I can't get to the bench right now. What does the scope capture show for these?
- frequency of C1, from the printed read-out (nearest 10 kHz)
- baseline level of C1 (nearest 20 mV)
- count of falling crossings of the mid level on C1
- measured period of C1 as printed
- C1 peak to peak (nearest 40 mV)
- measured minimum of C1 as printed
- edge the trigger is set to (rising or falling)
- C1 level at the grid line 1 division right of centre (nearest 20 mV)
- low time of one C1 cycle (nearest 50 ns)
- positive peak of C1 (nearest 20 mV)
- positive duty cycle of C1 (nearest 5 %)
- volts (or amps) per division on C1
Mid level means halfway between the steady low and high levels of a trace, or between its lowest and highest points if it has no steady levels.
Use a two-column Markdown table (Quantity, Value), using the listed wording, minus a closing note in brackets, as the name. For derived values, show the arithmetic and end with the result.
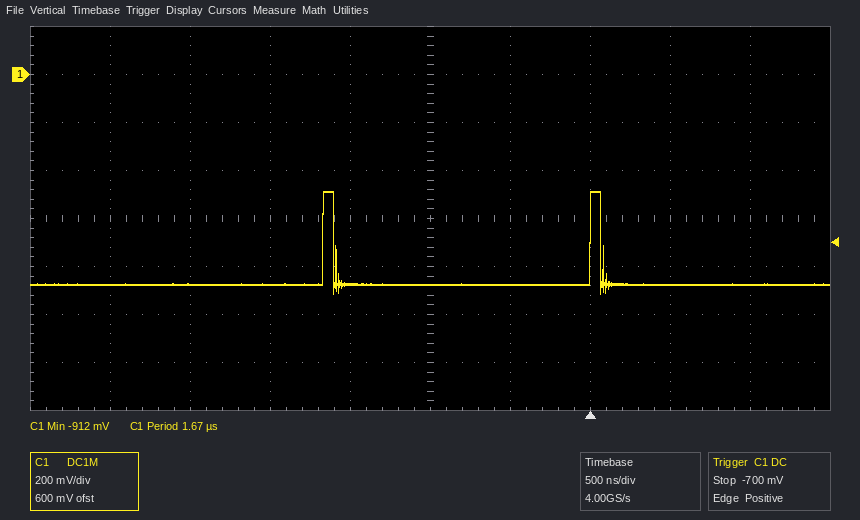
| Quantity | Value |
|---|---|
| frequency of C1, from the printed read-out | 1 / 1.67 µs ≈ 599 kHz, so 600 kHz to the nearest 10 kHz |
| baseline level of C1 | -880 mV |
| count of falling crossings of the mid level on C1 | 2 |
| measured period of C1 as printed | 1.67 µs |
| C1 peak to peak | 440 mV |
| measured minimum of C1 as printed | -912 mV |
| edge the trigger is set to | rising |
| C1 level at the grid line 1 division right of centre | -880 mV |
| low time of one C1 cycle | 1.60 µs |
| positive peak of C1 | -480 mV |
| positive duty cycle of C1 | 5 % |
| volts (or amps) per division on C1 | 200 mV |
